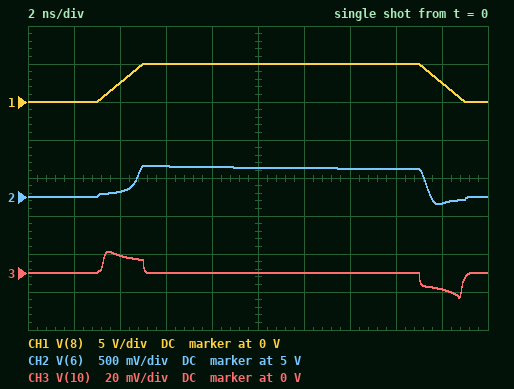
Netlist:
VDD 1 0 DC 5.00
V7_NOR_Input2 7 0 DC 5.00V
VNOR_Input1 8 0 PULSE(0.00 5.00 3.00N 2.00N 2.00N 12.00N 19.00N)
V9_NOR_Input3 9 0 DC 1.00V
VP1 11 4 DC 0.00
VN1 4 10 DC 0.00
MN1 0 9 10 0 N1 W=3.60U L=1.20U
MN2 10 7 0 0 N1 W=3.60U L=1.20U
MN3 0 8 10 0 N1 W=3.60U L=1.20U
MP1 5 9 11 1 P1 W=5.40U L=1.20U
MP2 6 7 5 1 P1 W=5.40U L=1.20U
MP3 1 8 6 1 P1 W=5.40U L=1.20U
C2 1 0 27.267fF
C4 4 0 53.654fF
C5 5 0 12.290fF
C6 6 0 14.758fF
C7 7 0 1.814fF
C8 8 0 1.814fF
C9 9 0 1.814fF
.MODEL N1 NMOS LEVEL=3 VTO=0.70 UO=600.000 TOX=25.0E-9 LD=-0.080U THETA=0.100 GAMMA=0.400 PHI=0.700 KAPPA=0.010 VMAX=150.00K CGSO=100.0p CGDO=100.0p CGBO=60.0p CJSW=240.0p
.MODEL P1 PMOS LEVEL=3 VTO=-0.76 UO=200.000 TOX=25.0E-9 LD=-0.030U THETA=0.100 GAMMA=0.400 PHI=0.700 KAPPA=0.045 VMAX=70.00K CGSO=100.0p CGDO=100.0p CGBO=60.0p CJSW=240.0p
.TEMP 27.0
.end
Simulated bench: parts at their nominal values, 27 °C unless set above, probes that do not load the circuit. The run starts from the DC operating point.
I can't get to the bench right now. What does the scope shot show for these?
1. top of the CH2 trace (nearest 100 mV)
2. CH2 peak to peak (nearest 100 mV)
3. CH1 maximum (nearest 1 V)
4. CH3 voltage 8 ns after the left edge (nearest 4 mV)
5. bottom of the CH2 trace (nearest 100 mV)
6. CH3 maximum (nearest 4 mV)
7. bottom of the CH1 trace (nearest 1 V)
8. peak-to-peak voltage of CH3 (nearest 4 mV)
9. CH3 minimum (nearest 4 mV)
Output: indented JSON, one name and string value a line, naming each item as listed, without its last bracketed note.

{
  "top of the CH2 trace": "5.4 V",
  "CH2 peak to peak": "500 mV",
  "CH1 maximum": "5 V",
  "CH3 voltage 8 ns after the left edge": "0 V",
  "bottom of the CH2 trace": "4.9 V",
  "CH3 maximum": "12 mV",
  "bottom of the CH1 trace": "0 V",
  "peak-to-peak voltage of CH3": "24 mV",
  "CH3 minimum": "-12 mV"
}
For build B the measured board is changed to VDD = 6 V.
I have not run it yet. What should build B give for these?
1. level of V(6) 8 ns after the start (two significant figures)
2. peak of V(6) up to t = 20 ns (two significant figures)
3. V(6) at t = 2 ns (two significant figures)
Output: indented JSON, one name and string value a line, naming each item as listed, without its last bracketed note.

{
  "level of V(6) 8 ns after the start": "5.9 V",
  "peak of V(6) up to t = 20 ns": "6.1 V",
  "V(6) at t = 2 ns": "6.0 V"
}
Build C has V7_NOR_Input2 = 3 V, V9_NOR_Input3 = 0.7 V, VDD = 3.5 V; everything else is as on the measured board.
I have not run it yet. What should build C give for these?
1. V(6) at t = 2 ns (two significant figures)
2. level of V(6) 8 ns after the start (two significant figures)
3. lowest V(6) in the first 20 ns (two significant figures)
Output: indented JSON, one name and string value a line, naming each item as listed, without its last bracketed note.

{
  "V(6) at t = 2 ns": "3.5 V",
  "level of V(6) 8 ns after the start": "3.8 V",
  "lowest V(6) in the first 20 ns": "3.4 V"
}
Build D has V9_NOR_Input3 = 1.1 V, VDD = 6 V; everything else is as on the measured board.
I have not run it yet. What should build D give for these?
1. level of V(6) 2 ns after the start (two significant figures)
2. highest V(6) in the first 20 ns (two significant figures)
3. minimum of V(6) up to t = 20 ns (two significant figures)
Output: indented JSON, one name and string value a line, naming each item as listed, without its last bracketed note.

{
  "level of V(6) 2 ns after the start": "6.0 V",
  "highest V(6) in the first 20 ns": "6.1 V",
  "minimum of V(6) up to t = 20 ns": "5.9 V"
}
